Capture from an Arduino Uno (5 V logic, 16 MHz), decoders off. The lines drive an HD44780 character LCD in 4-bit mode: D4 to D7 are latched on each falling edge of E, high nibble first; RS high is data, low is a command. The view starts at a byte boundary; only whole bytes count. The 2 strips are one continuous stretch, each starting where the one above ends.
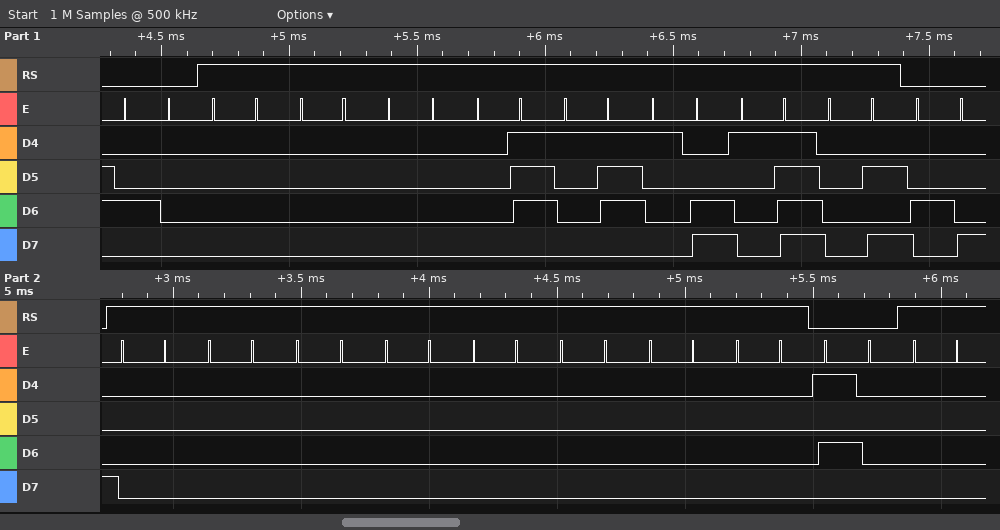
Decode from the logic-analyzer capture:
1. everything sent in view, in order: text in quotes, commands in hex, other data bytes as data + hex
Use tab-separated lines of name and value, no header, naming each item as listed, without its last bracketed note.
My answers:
everything sent in view, in order: text in quotes, commands in hex, other data bytes as data + hex	0x40 data 00 00 00 07 17 1C 1F 0A 0x48 data 00 00 00 00 00 00 00 00 0x50 data 00
